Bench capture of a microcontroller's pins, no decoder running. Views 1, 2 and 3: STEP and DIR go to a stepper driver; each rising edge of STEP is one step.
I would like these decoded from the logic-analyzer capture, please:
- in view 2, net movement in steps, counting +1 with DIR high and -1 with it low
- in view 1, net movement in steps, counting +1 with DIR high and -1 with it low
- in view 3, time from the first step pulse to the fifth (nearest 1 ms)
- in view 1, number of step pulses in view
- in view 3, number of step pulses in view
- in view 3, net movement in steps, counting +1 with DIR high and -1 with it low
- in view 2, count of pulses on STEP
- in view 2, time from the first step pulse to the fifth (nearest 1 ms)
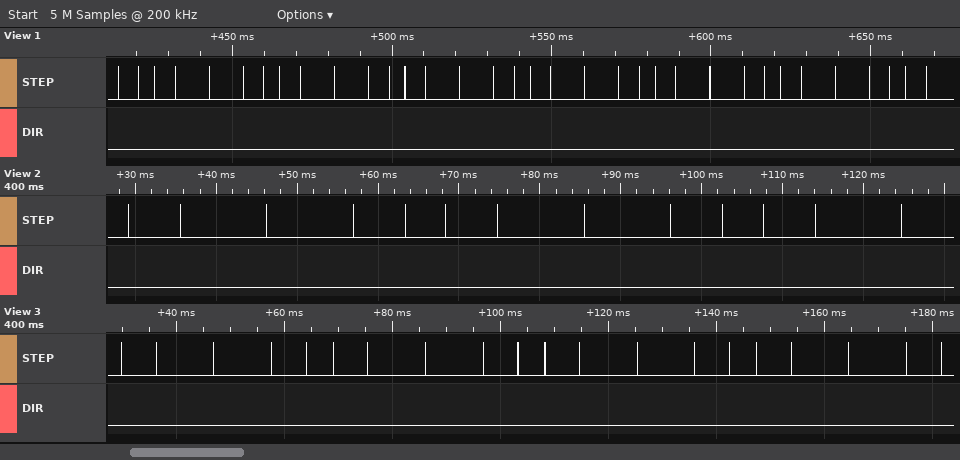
-13
-34
34 ms
34
20
-20
13
34 ms
